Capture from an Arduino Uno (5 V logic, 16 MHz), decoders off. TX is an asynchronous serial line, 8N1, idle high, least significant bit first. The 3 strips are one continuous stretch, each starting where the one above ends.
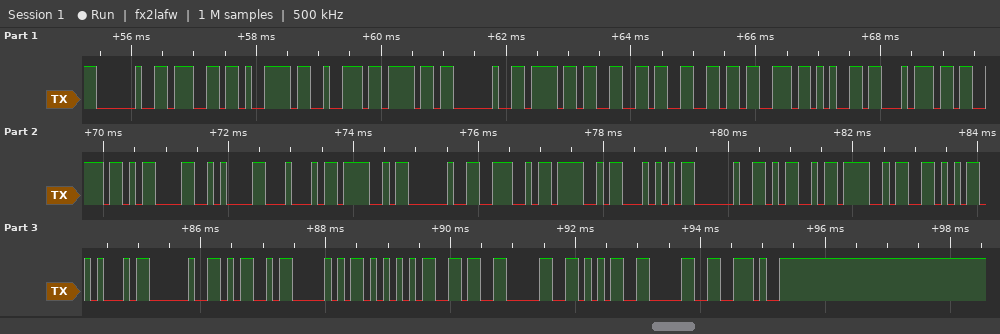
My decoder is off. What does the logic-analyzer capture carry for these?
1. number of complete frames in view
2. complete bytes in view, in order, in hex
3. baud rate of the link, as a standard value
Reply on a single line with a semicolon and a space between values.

35; 20 67 79 72 6F 20 6F 66 66 73 65 74 73 0D 0A 44 4F 20 4E 4F 54 20 4D 4F 56 45 20 4D 50 55 36 30 35 30 2E; 9600 baud
